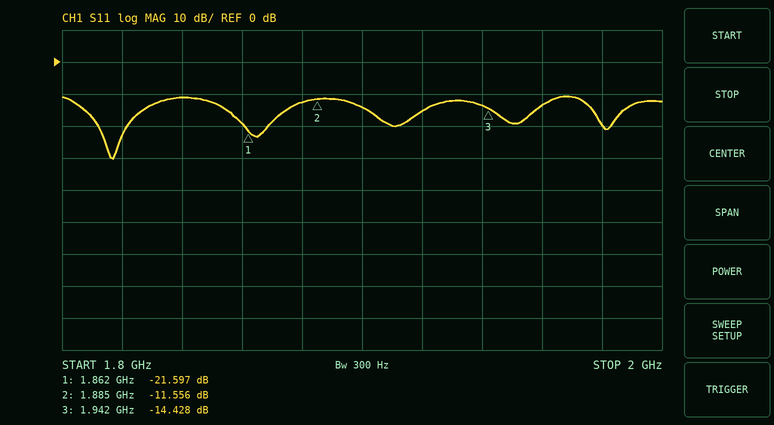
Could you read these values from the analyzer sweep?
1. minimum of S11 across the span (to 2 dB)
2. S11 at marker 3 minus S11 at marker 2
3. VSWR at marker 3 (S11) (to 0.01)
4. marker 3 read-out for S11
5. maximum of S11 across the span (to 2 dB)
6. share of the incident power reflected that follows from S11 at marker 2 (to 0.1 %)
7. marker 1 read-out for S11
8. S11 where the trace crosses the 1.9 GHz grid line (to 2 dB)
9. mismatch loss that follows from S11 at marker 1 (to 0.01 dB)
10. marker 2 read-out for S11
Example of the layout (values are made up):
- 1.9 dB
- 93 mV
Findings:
- -30 dB
- -2.872 dB
- 1.47
- -14.428 dB
- -10 dB
- 7.0 %
- -21.597 dB
- -14 dB
- 0.03 dB
- -11.556 dB
